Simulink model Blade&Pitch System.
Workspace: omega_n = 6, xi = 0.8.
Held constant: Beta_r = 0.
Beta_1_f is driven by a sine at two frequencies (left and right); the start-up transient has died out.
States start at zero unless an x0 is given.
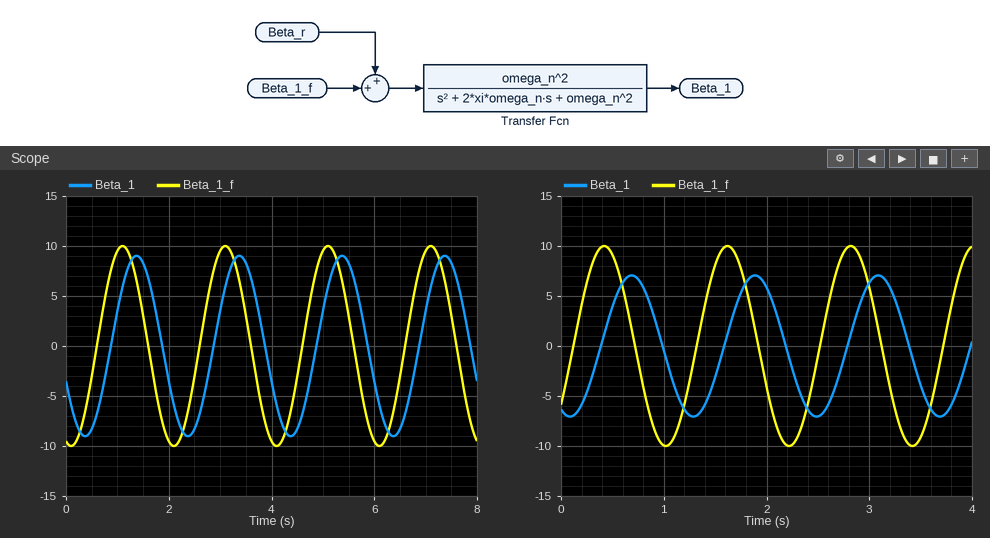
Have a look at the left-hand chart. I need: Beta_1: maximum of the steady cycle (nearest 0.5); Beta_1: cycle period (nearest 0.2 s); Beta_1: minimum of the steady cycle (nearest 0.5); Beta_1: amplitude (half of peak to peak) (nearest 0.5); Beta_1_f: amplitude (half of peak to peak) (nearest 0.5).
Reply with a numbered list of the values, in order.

1. 9.0
2. 2.0 s
3. -9.0
4. 9.0
5. 10.0
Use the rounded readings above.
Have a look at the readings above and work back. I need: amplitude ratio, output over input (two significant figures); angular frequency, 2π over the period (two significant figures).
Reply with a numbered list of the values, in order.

1. 0.90
2. 3.1 rad/s
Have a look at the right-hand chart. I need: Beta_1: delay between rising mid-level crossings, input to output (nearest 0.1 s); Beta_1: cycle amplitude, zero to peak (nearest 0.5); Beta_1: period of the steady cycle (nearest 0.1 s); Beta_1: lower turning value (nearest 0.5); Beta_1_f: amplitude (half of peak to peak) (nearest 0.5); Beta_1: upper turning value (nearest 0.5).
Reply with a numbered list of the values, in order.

1. 0.3 s
2. 7.0
3. 1.2 s
4. -7.0
5. 10.0
6. 7.0
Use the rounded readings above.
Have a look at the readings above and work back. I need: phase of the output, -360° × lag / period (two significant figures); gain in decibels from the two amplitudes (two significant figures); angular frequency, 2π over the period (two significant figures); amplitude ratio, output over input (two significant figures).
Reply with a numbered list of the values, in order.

1. -90°
2. -3.1 dB
3. 5.2 rad/s
4. 0.70
